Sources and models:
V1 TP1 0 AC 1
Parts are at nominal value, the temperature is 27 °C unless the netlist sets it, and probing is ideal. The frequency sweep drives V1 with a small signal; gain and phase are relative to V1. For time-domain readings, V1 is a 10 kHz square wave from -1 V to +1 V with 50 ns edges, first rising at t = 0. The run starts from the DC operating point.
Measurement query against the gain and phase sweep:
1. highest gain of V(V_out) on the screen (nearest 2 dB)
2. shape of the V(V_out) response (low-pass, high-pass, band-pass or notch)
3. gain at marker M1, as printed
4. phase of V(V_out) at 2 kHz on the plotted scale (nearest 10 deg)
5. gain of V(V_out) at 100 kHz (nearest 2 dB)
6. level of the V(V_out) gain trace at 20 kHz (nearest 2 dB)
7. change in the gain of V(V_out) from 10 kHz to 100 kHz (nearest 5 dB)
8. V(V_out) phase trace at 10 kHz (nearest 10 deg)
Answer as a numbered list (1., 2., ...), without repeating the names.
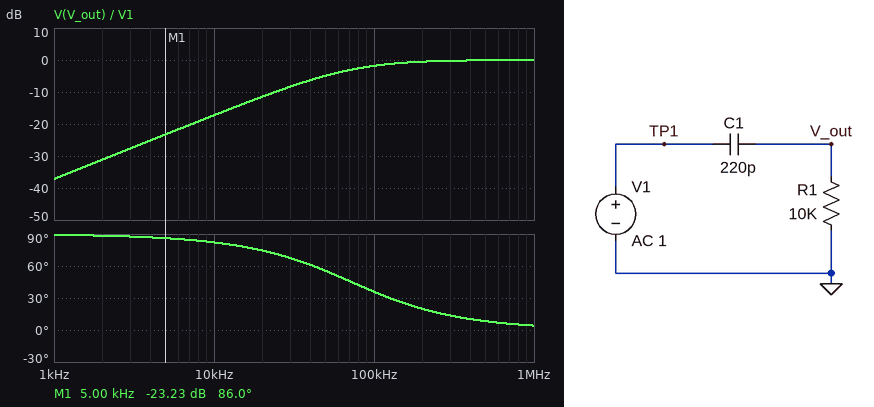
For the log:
1. 0 dB
2. high-pass
3. -23.23 dB
4. 90 deg
5. -2 dB
6. -12 dB
7. 15 dB
8. 80 deg
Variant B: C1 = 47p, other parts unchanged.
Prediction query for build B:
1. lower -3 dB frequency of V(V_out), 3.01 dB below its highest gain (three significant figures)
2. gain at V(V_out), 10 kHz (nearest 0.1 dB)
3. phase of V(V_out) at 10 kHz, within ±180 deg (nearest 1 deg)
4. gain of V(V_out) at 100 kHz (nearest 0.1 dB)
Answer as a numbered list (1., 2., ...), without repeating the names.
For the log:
1. 339 kHz
2. -30.6 dB
3. 88 deg
4. -11.0 dB
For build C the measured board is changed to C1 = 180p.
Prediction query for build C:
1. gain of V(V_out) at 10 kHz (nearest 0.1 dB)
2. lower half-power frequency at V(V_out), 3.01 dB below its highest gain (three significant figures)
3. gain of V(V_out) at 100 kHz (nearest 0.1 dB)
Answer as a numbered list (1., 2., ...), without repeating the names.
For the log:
1. -19.0 dB
2. 88.4 kHz
3. -2.5 dB
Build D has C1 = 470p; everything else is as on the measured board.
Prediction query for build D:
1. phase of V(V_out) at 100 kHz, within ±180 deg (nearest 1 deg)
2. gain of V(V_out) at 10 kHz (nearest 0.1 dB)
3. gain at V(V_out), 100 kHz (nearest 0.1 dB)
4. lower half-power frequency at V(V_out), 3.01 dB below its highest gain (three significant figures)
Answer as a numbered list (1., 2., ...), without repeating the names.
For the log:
1. 19 deg
2. -11.0 dB
3. -0.5 dB
4. 33.9 kHz
